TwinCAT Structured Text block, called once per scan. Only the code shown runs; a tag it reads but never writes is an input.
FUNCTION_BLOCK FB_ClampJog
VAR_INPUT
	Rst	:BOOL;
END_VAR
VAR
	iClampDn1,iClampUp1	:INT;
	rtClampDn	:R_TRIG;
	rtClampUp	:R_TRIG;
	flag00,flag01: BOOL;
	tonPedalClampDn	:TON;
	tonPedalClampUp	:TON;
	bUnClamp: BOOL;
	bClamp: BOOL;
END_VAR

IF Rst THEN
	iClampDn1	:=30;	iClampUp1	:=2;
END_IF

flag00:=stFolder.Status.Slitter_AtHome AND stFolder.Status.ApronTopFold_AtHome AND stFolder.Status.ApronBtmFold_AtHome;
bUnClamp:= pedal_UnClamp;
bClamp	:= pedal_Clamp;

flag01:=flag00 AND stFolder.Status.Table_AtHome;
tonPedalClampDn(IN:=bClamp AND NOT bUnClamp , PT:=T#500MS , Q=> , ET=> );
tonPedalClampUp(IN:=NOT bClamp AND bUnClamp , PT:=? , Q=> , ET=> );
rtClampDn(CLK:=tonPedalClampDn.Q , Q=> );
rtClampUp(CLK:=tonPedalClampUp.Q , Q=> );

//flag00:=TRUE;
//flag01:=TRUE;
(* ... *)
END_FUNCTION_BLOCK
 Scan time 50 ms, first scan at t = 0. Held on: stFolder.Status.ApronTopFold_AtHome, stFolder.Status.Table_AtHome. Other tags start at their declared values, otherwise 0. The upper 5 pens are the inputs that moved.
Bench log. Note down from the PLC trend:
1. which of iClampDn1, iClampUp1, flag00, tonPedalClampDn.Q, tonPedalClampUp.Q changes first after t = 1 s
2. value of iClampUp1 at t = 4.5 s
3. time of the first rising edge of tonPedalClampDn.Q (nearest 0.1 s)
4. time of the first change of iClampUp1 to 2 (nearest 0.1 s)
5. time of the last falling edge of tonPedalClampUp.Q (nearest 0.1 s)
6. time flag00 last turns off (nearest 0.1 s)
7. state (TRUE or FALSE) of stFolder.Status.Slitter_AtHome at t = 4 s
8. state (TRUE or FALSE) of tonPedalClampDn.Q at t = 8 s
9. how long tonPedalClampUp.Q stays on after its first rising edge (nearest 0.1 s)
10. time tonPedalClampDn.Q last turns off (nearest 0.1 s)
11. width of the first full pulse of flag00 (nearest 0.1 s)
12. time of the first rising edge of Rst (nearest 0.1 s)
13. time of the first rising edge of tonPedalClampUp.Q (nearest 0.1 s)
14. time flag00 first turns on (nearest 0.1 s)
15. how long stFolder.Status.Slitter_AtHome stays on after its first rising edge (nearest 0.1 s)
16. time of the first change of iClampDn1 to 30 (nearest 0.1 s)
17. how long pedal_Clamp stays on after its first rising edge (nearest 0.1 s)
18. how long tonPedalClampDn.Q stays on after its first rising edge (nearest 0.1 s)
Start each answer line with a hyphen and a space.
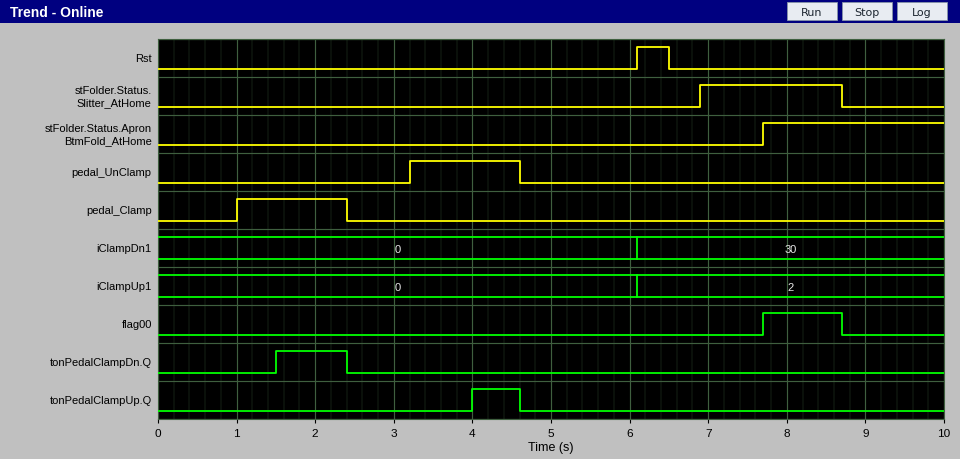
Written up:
- tonPedalClampDn.Q
- 0
- 1.5 s
- 6.1 s
- 4.6 s
- 8.7 s
- FALSE
- FALSE
- 0.6 s
- 2.4 s
- 1.0 s
- 6.1 s
- 4.0 s
- 7.7 s
- 1.8 s
- 6.1 s
- 1.4 s
- 0.9 s
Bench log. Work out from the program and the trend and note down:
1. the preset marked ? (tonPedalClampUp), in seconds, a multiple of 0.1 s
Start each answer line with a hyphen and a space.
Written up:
- 0.8 s
